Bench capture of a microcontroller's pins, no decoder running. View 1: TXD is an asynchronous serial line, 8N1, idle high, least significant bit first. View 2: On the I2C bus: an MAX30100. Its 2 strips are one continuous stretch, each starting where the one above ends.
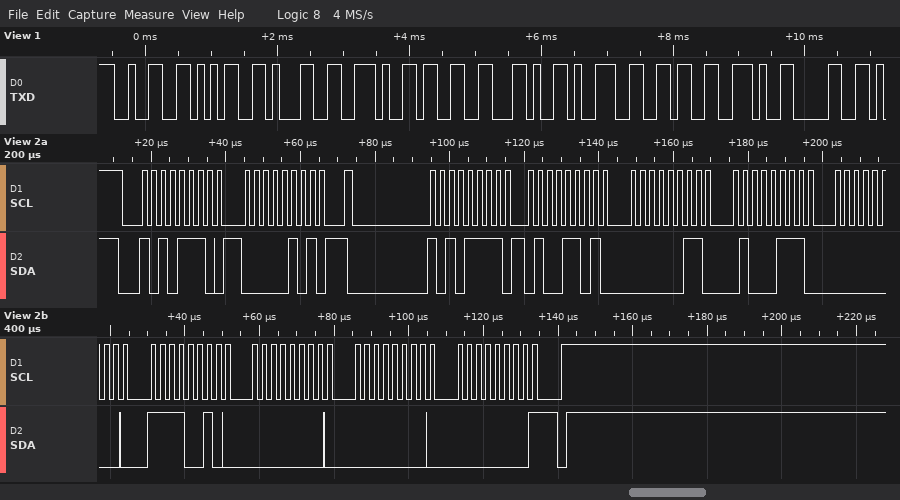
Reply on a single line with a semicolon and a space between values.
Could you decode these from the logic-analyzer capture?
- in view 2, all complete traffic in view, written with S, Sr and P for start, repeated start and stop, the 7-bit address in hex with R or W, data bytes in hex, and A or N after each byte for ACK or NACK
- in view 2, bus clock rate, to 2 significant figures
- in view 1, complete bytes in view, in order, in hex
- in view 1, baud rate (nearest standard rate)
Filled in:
S 57W A 05 A Sr 57R A 4D A 03 A 47 A 00 A F2 A 00 A 00 A 00 N P; 400 kHz; 0x32 0x35 0x31 0x2E 0x33 0x2C 0x39 0x36 0x2E 0x30; 9600 baud
